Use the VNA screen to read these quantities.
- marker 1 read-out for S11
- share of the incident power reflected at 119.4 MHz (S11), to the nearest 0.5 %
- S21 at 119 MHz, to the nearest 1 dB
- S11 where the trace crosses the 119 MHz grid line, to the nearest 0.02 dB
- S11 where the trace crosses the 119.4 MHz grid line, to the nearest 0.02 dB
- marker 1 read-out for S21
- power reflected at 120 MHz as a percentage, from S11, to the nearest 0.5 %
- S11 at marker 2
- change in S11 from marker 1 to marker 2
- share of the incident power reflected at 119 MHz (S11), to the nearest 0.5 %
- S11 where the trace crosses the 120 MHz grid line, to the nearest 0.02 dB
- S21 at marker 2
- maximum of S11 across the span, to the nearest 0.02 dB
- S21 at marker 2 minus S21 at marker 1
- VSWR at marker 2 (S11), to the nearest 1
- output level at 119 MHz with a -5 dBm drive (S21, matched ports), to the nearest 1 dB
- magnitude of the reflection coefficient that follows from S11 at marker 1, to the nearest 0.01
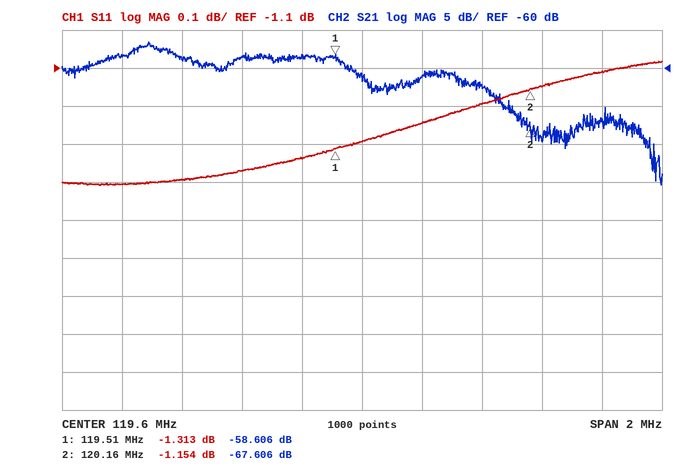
-1.313 dB
73.5 %
-59 dB
-1.40 dB
-1.34 dB
-58.606 dB
76.0 %
-1.154 dB
0.159 dB
72.5 %
-1.20 dB
-67.606 dB
-1.08 dB
-9.000 dB
15
-64 dBm
0.86
